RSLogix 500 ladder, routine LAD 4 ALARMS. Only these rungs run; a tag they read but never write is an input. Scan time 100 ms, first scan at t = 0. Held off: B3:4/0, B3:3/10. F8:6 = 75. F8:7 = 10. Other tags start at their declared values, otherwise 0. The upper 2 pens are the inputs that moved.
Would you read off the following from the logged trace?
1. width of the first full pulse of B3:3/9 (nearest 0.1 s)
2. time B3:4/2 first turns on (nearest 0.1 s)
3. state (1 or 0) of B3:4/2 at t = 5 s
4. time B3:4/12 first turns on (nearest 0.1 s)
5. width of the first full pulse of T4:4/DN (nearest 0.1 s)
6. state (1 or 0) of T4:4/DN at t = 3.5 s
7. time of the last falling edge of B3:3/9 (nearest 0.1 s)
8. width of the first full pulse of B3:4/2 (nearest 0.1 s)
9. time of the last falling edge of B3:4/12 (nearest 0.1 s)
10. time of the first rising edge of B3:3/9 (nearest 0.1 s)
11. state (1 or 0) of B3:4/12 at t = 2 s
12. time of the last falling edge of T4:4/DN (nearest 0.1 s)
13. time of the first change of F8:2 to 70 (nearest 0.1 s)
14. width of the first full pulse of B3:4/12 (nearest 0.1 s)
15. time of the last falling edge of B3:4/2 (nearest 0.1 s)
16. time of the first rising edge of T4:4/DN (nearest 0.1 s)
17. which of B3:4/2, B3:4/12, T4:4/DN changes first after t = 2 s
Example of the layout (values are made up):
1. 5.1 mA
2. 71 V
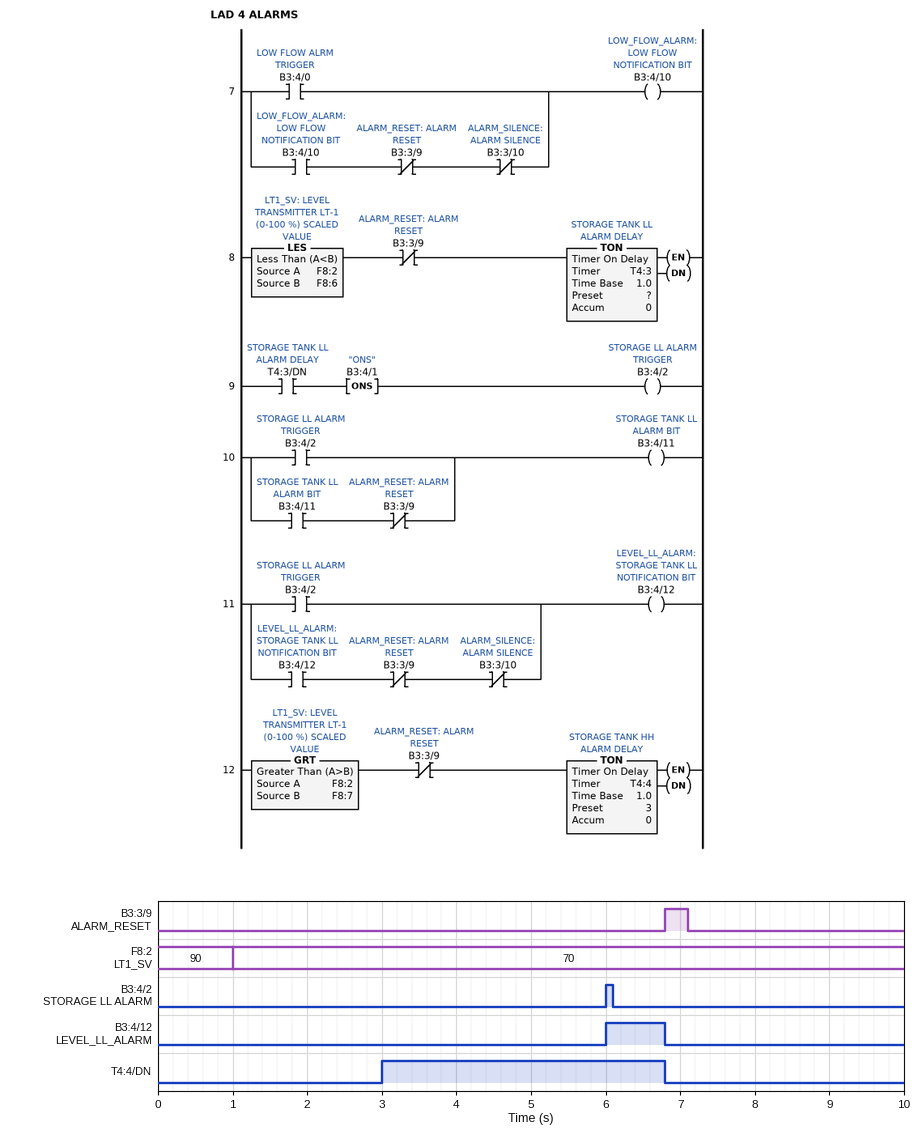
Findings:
1. 0.3 s
2. 6.0 s
3. 0
4. 6.0 s
5. 3.8 s
6. 1
7. 7.1 s
8. 0.1 s
9. 6.8 s
10. 6.8 s
11. 0
12. 6.8 s
13. 1.0 s
14. 0.8 s
15. 6.1 s
16. 3.0 s
17. T4:4/DN
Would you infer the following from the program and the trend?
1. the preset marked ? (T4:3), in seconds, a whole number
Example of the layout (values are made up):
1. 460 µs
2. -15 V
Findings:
1. 5 s
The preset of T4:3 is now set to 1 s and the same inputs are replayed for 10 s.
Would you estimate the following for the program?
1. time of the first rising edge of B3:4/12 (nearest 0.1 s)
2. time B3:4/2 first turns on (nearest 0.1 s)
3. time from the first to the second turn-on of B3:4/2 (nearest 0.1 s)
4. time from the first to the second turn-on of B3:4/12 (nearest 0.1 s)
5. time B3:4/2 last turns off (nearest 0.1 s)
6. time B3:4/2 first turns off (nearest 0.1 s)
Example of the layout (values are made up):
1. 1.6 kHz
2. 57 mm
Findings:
1. 2.0 s
2. 2.0 s
3. 6.1 s
4. 6.1 s
5. 8.2 s
6. 2.1 s
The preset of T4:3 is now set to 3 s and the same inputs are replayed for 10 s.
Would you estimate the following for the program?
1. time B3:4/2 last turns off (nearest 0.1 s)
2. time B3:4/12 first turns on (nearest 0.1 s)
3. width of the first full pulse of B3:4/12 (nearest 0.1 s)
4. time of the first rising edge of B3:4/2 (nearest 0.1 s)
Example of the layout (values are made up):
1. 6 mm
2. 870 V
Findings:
1. 4.1 s
2. 4.0 s
3. 2.8 s
4. 4.0 s
